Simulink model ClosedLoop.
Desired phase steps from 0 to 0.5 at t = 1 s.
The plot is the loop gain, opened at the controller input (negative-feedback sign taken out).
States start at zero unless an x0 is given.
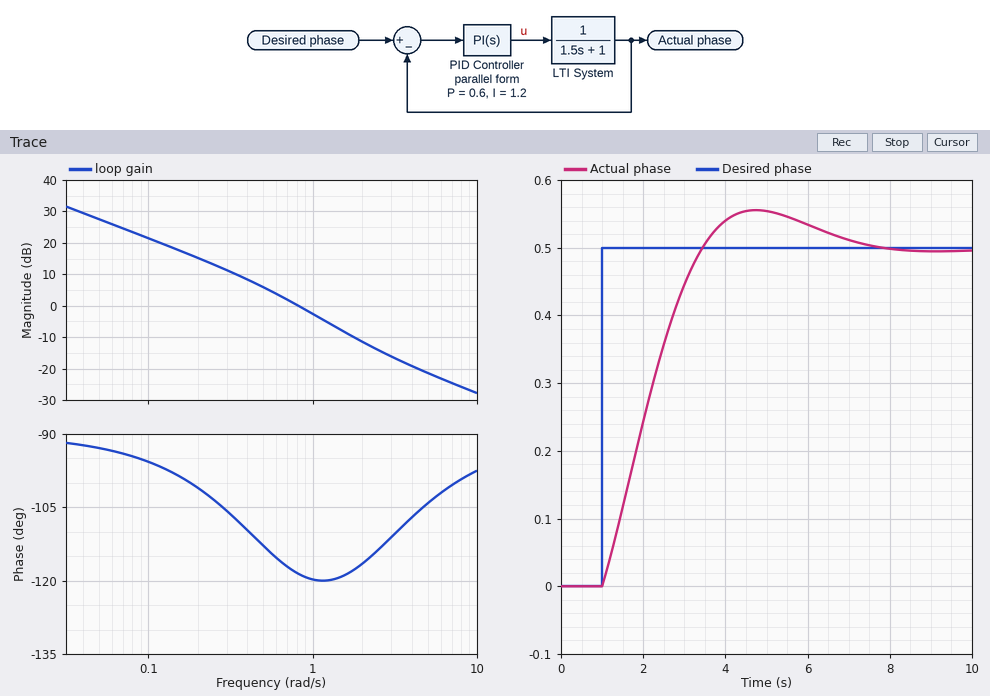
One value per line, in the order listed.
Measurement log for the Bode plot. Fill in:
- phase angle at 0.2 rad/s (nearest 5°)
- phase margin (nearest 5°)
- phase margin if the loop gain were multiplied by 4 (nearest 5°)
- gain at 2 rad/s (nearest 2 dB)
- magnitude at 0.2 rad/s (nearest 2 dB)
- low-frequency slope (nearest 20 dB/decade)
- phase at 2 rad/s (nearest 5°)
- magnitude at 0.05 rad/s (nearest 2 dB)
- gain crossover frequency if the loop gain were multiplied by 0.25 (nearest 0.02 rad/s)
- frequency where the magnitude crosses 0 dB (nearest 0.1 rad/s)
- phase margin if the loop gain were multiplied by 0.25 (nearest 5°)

-100°
60°
65°
-12 dB
16 dB
-20 dB/decade
-115°
28 dB
0.28 rad/s
0.8 rad/s
75°
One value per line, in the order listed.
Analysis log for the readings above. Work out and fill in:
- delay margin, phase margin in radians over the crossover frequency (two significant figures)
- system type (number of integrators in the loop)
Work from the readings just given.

1.3 s
1
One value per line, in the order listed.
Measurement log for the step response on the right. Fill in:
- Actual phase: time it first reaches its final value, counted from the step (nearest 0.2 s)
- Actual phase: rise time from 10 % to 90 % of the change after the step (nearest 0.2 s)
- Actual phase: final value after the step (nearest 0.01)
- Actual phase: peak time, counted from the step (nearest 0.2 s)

2.4 s
1.8 s
0.50
3.8 s
